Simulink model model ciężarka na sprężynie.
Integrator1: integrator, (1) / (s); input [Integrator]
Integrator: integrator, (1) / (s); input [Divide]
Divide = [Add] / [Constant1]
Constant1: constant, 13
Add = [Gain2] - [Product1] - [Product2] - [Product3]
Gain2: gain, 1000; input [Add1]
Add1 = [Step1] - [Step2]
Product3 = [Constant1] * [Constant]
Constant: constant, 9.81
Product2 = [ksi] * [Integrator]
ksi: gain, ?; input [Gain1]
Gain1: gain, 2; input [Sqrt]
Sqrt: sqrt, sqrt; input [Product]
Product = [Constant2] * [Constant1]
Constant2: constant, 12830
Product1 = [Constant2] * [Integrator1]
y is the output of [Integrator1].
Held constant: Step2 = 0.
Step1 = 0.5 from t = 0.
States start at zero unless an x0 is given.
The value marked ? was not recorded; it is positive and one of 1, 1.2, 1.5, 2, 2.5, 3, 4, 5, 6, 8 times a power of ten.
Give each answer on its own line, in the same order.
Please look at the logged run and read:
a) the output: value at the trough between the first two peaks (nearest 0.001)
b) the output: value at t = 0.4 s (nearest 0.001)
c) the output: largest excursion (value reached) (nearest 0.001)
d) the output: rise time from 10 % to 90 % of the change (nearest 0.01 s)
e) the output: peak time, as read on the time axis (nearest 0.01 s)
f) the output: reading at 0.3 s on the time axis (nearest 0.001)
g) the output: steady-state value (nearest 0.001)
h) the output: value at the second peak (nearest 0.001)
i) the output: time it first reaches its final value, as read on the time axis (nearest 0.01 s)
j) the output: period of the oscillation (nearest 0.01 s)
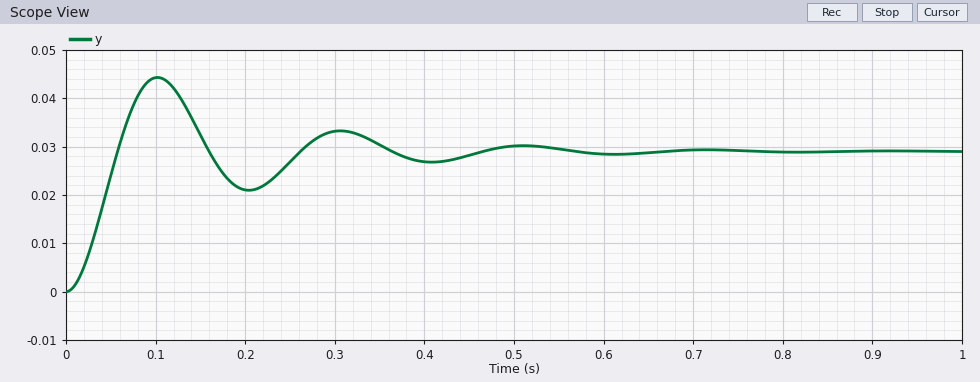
0.021
0.027
0.044
0.04 s
0.10 s
0.033
0.029
0.033
0.06 s
0.20 s
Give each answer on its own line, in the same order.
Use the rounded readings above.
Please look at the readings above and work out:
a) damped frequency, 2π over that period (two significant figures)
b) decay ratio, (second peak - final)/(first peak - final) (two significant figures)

31 rad/s
0.27
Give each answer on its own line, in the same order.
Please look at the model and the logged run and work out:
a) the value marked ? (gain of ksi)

0.2
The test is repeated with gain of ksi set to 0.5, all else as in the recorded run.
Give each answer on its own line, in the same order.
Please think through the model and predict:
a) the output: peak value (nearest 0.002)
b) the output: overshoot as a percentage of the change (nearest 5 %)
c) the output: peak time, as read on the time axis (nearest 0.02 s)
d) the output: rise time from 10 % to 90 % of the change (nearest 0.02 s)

0.034
15 %
0.12 s
0.06 s
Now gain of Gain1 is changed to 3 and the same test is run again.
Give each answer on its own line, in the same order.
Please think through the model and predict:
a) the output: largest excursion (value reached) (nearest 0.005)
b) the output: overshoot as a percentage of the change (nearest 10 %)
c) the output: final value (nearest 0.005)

0.040
40 %
0.030
